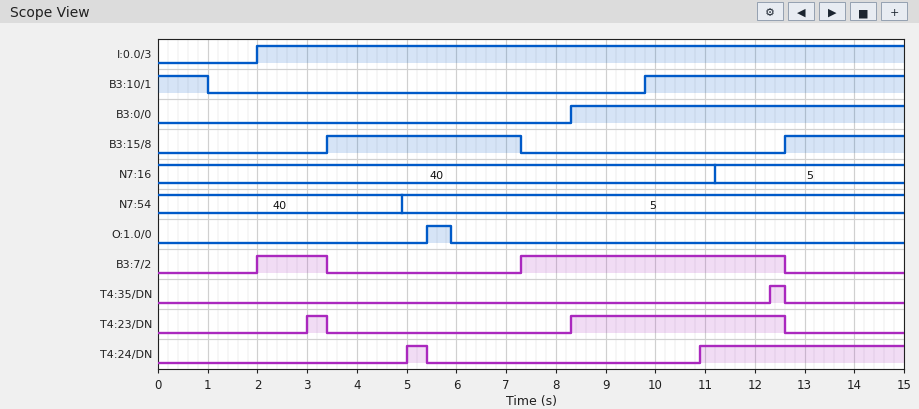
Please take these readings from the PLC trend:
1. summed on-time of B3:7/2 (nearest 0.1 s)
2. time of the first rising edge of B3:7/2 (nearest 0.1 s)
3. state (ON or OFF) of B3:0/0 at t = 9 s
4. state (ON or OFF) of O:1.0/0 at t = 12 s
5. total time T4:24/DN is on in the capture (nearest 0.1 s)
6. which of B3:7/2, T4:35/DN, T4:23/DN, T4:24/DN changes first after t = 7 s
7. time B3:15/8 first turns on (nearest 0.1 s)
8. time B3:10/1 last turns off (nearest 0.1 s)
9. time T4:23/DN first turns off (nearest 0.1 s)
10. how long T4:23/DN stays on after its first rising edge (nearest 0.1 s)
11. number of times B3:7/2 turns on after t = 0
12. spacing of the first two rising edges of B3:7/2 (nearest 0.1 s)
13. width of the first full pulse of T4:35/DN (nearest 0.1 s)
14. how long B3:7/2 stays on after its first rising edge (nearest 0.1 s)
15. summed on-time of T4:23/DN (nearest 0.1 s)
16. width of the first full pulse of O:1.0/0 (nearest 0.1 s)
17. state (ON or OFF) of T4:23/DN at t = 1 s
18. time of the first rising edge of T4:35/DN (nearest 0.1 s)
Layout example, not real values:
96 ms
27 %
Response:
6.7 s
2.0 s
ON
OFF
4.5 s
B3:7/2
3.4 s
1.0 s
3.4 s
0.4 s
2
5.3 s
0.3 s
1.4 s
4.7 s
0.5 s
OFF
12.3 s
